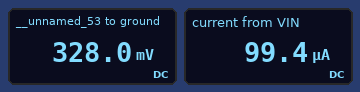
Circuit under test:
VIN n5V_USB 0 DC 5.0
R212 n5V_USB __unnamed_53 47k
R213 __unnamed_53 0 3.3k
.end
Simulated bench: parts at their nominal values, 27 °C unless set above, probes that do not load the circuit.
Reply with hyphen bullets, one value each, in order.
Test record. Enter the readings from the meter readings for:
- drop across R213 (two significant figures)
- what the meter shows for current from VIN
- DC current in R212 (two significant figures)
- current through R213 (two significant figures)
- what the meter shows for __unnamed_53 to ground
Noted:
- 330 mV
- 99.4 µA
- 99 µA
- 99 µA
- 328.0 mV
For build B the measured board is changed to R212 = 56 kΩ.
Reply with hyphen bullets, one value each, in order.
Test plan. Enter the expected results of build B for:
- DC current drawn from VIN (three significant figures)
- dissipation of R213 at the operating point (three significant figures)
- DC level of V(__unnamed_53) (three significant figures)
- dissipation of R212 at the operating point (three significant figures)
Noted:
- 84.3 µA
- 23.5 µW
- 278 mV
- 398 µW
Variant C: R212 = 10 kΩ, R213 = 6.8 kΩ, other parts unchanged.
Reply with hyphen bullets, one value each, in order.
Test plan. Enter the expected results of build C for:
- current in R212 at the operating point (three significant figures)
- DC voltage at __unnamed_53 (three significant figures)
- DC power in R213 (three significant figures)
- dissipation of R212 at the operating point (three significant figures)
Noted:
- 298 µA
- 2.02 V
- 602 µW
- 886 µW
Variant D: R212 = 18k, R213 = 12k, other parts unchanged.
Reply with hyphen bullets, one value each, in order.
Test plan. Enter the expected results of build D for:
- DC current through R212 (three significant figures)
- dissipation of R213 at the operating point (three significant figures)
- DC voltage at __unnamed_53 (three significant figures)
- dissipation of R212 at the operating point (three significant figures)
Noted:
- 167 µA
- 333 µW
- 2.00 V
- 500 µW
